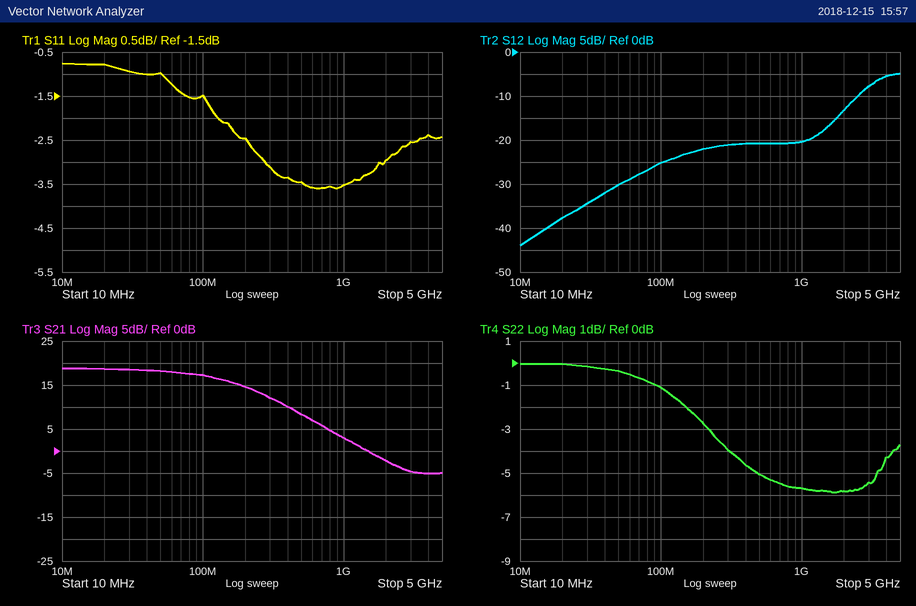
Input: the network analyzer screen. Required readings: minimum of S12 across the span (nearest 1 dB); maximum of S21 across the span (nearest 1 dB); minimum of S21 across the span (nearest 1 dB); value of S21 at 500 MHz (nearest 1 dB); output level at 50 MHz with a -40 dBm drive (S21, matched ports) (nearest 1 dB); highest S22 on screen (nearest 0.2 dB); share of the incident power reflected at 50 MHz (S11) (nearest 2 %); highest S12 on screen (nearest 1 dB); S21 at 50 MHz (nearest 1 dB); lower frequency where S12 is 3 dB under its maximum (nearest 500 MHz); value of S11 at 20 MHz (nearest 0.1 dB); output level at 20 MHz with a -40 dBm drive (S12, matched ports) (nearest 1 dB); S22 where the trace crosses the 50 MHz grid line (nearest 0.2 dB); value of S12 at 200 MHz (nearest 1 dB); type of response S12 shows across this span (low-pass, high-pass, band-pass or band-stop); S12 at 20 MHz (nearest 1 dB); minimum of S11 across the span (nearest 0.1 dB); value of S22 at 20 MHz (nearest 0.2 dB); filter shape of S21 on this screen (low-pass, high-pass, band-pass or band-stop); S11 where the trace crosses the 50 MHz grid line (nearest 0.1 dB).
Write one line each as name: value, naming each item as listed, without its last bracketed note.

minimum of S12 across the span: -44 dB
maximum of S21 across the span: 19 dB
minimum of S21 across the span: -5 dB
value of S21 at 500 MHz: 8 dB
output level at 50 MHz with a -40 dBm drive (S21, matched ports): -22 dBm
highest S22 on screen: 0.0 dB
share of the incident power reflected at 50 MHz (S11): 80 %
highest S12 on screen: -5 dB
S21 at 50 MHz: 18 dB
lower frequency where S12 is 3 dB under its maximum: 3.0 GHz
value of S11 at 20 MHz: -0.8 dB
output level at 20 MHz with a -40 dBm drive (S12, matched ports): -78 dBm
S22 where the trace crosses the 50 MHz grid line: -0.4 dB
value of S12 at 200 MHz: -22 dB
type of response S12 shows across this span: high-pass
S12 at 20 MHz: -38 dB
minimum of S11 across the span: -3.6 dB
value of S22 at 20 MHz: 0.0 dB
filter shape of S21 on this screen: low-pass
S11 where the trace crosses the 50 MHz grid line: -1.0 dB
